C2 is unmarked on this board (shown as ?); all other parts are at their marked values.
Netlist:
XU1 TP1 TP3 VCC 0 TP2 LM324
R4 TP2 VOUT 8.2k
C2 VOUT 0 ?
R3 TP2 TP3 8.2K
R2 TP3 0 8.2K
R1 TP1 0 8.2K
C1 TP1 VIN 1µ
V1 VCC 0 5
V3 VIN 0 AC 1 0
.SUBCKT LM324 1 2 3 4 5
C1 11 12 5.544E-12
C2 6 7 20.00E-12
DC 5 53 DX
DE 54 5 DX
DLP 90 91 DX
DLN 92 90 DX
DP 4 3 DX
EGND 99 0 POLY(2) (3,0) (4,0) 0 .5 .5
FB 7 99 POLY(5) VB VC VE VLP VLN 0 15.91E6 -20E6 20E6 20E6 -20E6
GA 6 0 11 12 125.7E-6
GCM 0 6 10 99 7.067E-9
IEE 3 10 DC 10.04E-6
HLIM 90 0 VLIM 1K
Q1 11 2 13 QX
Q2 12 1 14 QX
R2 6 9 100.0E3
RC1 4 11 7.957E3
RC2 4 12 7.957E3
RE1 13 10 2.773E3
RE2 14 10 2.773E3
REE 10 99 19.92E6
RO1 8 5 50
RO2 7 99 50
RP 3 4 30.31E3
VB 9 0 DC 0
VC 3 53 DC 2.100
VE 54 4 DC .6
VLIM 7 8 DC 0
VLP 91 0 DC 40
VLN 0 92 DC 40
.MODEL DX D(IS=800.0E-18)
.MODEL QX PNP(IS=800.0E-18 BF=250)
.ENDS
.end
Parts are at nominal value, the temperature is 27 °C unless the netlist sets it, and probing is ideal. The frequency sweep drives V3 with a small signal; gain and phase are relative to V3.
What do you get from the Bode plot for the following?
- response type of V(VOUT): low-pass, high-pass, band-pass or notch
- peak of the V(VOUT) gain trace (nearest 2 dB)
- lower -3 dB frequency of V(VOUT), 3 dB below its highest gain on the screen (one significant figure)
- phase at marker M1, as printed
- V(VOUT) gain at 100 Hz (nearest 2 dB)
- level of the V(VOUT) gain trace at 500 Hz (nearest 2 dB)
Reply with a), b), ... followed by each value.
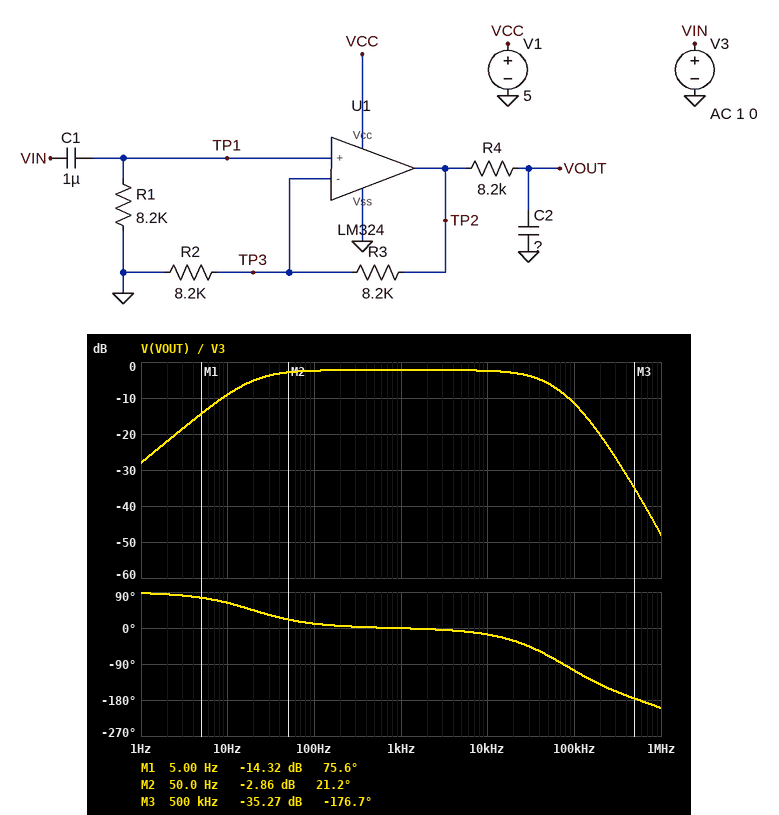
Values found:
a) band-pass
b) -2 dB
c) 20 Hz
d) 75.6 deg
e) -2 dB
f) -2 dB
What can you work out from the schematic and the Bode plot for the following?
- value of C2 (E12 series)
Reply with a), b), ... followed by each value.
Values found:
a) 390 pF
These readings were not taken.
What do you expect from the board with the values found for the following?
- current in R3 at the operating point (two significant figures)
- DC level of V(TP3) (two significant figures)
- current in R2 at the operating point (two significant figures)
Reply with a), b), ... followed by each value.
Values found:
a) 2.5 µA
b) 20 mV
c) 2.5 µA
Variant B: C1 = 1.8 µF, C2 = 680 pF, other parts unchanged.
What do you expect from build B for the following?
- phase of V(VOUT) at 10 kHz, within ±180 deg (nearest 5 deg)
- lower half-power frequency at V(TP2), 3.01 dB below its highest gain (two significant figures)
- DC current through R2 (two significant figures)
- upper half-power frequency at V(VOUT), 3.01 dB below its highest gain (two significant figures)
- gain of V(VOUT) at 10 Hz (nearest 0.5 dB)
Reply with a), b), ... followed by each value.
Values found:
a) -25 deg
b) 11 Hz
c) 2.5 µA
d) 27 kHz
e) -5.5 dB
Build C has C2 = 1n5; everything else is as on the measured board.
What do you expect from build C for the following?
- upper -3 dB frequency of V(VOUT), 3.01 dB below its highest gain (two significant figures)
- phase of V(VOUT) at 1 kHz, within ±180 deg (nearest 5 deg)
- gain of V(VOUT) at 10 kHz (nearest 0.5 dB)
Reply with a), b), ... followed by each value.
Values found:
a) 13 kHz
b) -5 deg
c) -4.5 dB
